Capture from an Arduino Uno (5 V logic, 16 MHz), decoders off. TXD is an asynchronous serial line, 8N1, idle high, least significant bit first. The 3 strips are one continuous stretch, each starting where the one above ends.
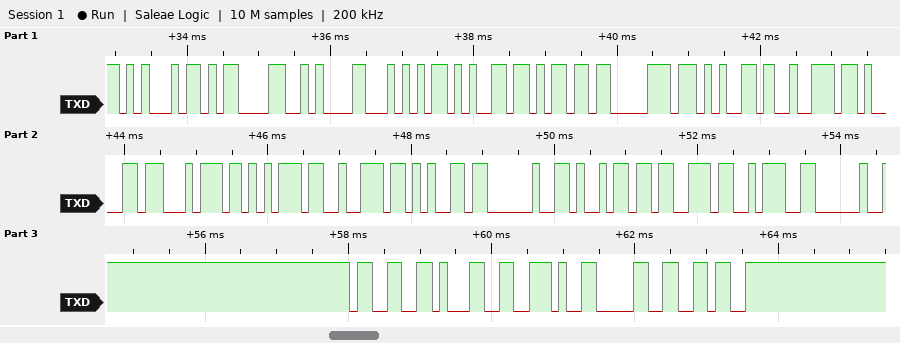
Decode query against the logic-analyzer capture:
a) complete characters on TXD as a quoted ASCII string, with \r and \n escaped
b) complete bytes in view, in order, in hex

"E\r\nTemperature is: 31.06"
45 0D 0A 54 65 6D 70 65 72 61 74 75 72 65 20 69 73 3A 20 33 31 2E 30 36
